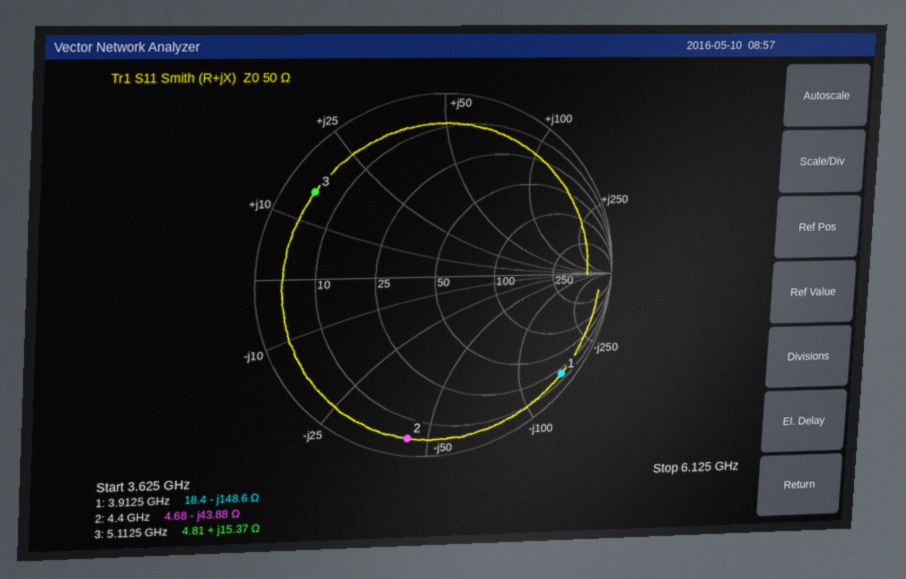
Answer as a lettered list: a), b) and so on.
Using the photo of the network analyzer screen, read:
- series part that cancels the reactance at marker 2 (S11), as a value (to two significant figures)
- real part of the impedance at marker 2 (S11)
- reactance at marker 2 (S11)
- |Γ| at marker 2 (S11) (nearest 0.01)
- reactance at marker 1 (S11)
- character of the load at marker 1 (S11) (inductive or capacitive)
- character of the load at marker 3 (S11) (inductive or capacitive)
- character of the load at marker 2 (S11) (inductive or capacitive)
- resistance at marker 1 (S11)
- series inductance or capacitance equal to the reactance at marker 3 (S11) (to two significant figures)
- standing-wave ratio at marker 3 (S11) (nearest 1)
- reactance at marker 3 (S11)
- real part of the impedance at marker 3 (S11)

a) 1.6 nH
b) 4.68 Ω
c) -43.88 Ω
d) 0.90
e) -148.6 Ω
f) capacitive
g) inductive
h) capacitive
i) 18.4 Ω
j) 480 pH
k) 11
l) +15.37 Ω
m) 4.81 Ω
